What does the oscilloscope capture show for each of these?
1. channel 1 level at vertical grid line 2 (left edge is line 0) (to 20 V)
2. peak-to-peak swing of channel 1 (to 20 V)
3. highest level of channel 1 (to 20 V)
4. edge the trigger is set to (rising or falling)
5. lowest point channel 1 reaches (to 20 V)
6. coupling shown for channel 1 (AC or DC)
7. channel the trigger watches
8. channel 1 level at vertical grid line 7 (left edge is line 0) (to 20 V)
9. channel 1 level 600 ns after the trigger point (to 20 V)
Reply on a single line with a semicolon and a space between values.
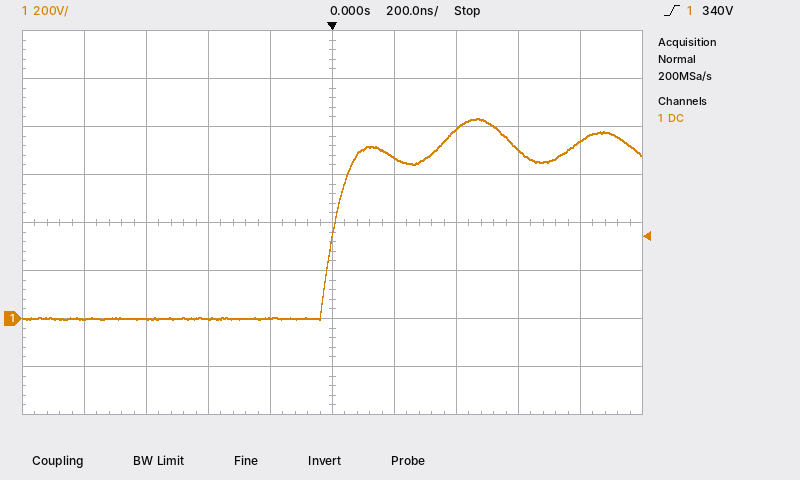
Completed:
0 V; 840 V; 840 V; rising; 0 V; DC; channel 1; 780 V; 700 V
